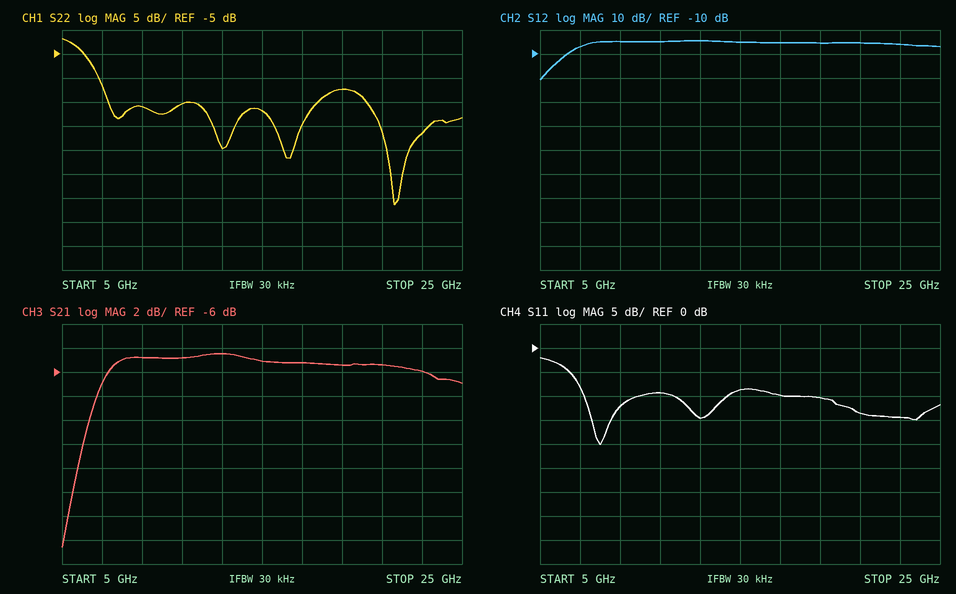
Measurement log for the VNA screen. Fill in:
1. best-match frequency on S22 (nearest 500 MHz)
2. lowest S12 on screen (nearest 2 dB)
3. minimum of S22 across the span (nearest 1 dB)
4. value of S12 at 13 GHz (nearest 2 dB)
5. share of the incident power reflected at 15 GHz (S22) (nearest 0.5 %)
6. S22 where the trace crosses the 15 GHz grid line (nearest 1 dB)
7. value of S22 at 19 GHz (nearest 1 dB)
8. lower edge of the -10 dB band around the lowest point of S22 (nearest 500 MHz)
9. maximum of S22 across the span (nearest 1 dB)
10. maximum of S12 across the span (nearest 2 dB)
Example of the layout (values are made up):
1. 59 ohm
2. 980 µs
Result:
1. 21.5 GHz
2. -20 dB
3. -36 dB
4. -4 dB
5. 2.0 %
6. -17 dB
7. -12 dB
8. 7.0 GHz
9. -2 dB
10. -4 dB
